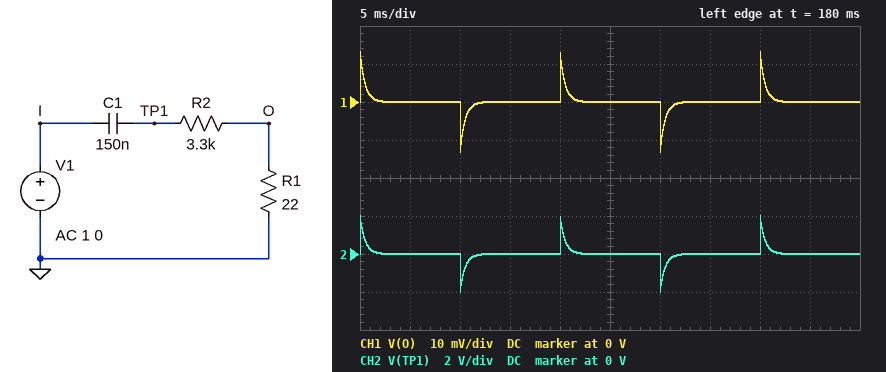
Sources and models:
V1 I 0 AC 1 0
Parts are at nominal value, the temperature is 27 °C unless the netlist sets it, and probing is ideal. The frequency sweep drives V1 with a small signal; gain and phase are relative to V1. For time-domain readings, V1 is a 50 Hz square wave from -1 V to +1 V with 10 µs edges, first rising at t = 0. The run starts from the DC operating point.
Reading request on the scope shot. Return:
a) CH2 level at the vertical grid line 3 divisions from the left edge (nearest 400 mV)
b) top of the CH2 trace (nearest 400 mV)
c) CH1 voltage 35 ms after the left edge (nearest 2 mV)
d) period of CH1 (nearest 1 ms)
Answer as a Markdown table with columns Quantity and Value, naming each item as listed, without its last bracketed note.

| Quantity | Value |
|---|---|
| CH2 level at the vertical grid line 3 divisions from the left edge | 0 V |
| top of the CH2 trace | 2.0 V |
| CH1 voltage 35 ms after the left edge | 0 V |
| period of CH1 | 20 ms |
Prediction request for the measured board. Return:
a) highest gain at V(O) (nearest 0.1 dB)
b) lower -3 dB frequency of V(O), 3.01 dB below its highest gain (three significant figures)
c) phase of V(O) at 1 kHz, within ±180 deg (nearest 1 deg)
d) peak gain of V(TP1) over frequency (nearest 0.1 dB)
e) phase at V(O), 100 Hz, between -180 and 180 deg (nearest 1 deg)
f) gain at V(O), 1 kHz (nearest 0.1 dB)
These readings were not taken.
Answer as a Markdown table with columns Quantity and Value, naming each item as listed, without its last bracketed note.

| Quantity | Value |
|---|---|
| highest gain at V(O) | -43.6 dB |
| lower -3 dB frequency of V(O), 3.01 dB below its highest gain | 319 Hz |
| phase of V(O) at 1 kHz, within ±180 deg | 18 deg |
| peak gain of V(TP1) over frequency | 0 dB |
| phase at V(O), 100 Hz, between -180 and 180 deg | 73 deg |
| gain at V(O), 1 kHz | -44.0 dB |
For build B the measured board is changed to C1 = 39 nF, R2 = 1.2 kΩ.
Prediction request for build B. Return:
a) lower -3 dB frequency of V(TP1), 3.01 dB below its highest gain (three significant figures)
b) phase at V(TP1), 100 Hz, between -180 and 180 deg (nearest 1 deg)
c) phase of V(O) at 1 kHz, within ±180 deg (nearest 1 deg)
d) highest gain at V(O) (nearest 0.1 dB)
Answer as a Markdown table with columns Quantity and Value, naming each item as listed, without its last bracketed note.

| Quantity | Value |
|---|---|
| lower -3 dB frequency of V(TP1), 3.01 dB below its highest gain | 3.34 kHz |
| phase at V(TP1), 100 Hz, between -180 and 180 deg | 88 deg |
| phase of V(O) at 1 kHz, within ±180 deg | 73 deg |
| highest gain at V(O) | -34.9 dB |
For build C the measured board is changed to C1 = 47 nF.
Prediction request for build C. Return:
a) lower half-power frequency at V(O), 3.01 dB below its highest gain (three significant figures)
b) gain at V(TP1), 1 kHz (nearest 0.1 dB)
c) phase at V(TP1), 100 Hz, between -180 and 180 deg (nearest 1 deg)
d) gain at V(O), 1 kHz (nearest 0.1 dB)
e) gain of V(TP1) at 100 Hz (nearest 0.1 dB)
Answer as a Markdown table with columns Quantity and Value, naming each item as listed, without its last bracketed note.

| Quantity | Value |
|---|---|
| lower half-power frequency at V(O), 3.01 dB below its highest gain | 1.02 kHz |
| gain at V(TP1), 1 kHz | -3.1 dB |
| phase at V(TP1), 100 Hz, between -180 and 180 deg | 84 deg |
| gain at V(O), 1 kHz | -46.7 dB |
| gain of V(TP1) at 100 Hz | -20.2 dB |
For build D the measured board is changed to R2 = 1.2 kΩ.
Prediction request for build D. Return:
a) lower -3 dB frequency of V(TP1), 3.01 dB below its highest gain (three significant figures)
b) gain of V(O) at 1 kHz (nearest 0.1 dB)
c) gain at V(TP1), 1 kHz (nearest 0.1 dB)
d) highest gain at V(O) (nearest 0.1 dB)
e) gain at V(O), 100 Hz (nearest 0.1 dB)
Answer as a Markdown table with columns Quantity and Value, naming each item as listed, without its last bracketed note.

| Quantity | Value |
|---|---|
| lower -3 dB frequency of V(TP1), 3.01 dB below its highest gain | 868 Hz |
| gain of V(O) at 1 kHz | -37.3 dB |
| gain at V(TP1), 1 kHz | -2.4 dB |
| highest gain at V(O) | -34.9 dB |
| gain at V(O), 100 Hz | -53.7 dB |
